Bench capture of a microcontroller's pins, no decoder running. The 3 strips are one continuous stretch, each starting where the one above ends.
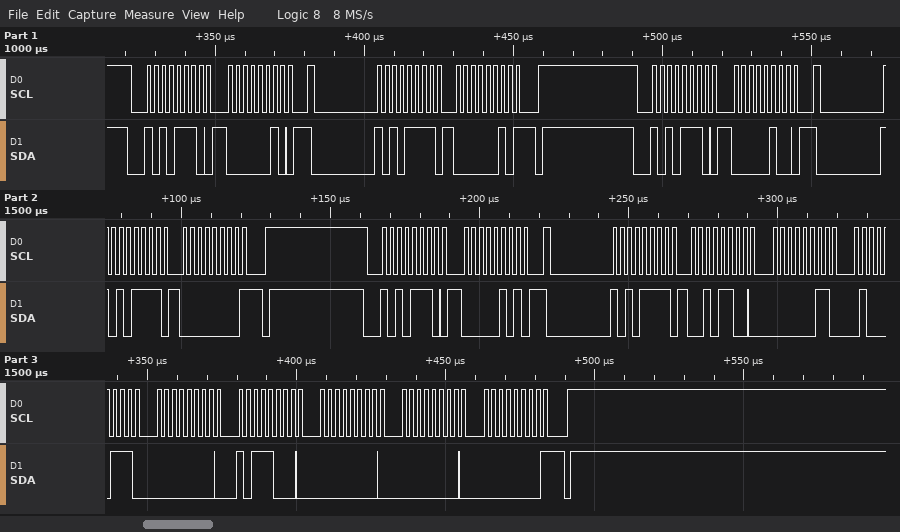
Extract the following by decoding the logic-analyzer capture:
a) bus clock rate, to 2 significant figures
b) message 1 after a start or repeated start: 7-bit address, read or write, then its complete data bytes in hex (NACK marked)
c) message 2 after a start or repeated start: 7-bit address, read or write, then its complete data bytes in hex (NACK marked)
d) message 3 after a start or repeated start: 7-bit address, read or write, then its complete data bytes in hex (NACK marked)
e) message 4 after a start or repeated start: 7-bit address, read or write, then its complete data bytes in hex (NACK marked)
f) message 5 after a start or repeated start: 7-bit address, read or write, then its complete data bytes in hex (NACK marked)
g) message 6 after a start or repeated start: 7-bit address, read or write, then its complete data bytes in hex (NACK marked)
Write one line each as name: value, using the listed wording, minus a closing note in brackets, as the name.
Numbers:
bus clock rate, to 2 significant figures: 400 kHz
message 1 after a start or repeated start: 7-bit address, read or write, then its complete data bytes in hex: 0x57 write: 02
message 2 after a start or repeated start: 7-bit address, read or write, then its complete data bytes in hex: 0x57 read: 02 NACK
message 3 after a start or repeated start: 7-bit address, read or write, then its complete data bytes in hex: 0x57 write: 04
message 4 after a start or repeated start: 7-bit address, read or write, then its complete data bytes in hex: 0x57 read: 00 NACK
message 5 after a start or repeated start: 7-bit address, read or write, then its complete data bytes in hex: 0x57 write: 05
message 6 after a start or repeated start: 7-bit address, read or write, then its complete data bytes in hex: 0x57 read: 2C 03 47 00 B8 00 00 00 NACK
